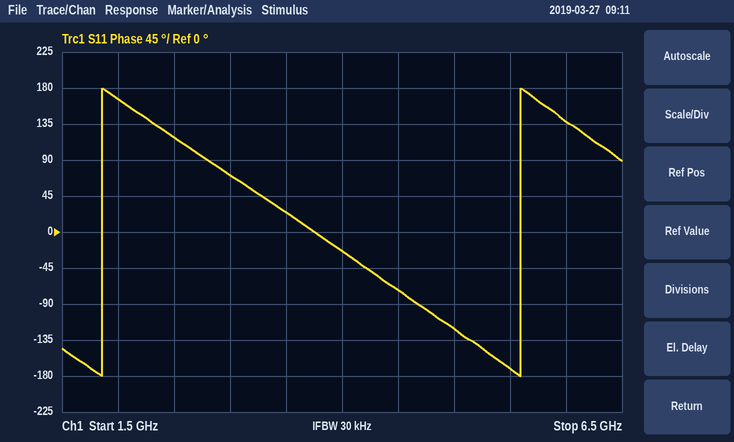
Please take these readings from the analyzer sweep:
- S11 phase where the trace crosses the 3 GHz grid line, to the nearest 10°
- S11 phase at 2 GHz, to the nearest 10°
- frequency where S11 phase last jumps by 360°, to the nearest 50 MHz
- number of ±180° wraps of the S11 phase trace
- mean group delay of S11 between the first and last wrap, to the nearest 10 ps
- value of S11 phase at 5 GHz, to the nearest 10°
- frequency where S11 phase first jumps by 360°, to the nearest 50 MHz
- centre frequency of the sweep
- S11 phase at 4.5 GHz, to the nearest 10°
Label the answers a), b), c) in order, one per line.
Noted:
a) 70°
b) 170°
c) 5.60 GHz
d) 2
e) 270 ps
f) -120°
g) 1.85 GHz
h) 4 GHz
i) -70°
